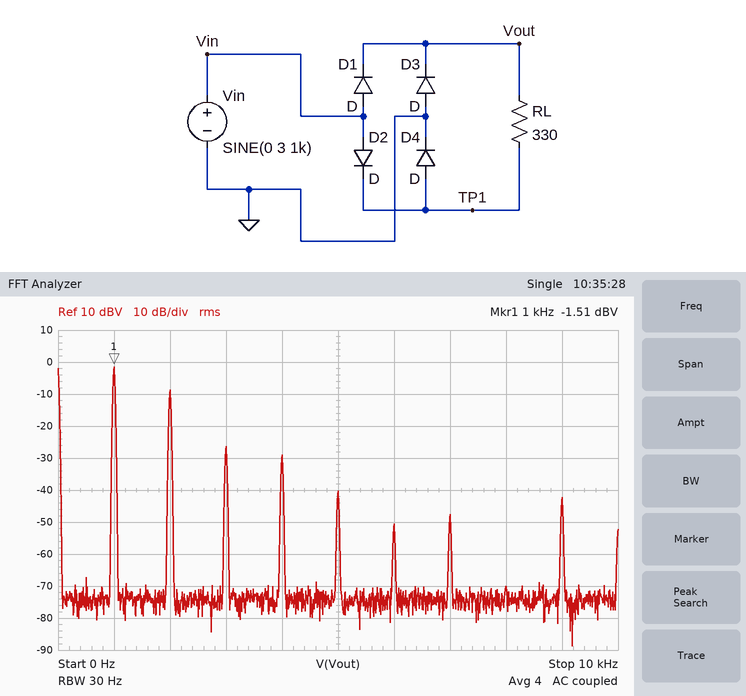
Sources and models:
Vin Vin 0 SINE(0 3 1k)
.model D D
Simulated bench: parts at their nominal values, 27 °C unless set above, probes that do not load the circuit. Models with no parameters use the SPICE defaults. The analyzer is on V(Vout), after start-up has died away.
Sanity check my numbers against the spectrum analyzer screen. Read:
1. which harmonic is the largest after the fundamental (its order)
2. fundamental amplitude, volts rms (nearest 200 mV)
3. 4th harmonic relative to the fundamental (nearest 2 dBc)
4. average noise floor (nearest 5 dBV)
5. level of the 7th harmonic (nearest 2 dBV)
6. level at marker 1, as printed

2
800 mV
-28 dBc
-75 dBV
-48 dBV
-1.51 dBV
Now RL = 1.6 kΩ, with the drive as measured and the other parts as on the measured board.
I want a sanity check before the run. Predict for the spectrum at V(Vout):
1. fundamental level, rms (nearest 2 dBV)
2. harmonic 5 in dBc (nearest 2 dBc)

-2 dBV
-38 dBc
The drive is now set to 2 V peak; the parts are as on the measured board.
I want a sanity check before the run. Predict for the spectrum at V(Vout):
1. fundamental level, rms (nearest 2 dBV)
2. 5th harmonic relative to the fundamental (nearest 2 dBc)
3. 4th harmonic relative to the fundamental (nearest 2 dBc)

-6 dBV
-36 dBc
-36 dBc
